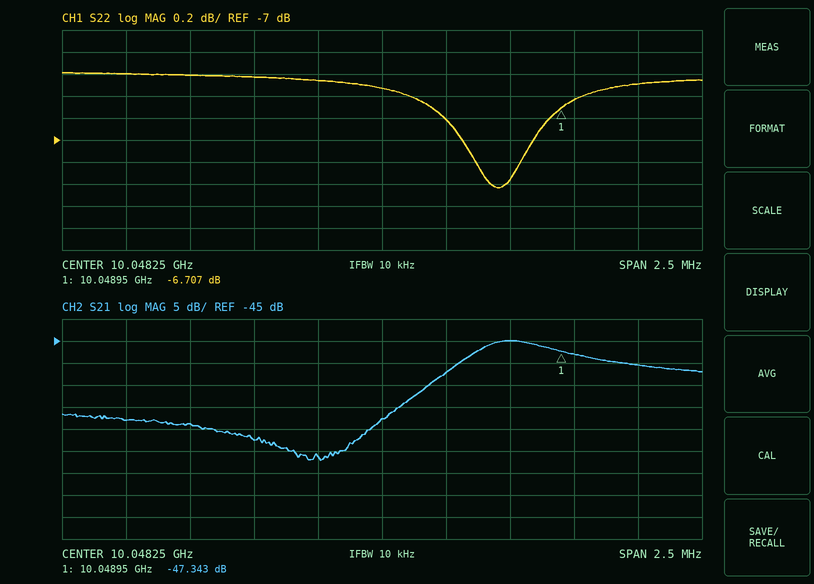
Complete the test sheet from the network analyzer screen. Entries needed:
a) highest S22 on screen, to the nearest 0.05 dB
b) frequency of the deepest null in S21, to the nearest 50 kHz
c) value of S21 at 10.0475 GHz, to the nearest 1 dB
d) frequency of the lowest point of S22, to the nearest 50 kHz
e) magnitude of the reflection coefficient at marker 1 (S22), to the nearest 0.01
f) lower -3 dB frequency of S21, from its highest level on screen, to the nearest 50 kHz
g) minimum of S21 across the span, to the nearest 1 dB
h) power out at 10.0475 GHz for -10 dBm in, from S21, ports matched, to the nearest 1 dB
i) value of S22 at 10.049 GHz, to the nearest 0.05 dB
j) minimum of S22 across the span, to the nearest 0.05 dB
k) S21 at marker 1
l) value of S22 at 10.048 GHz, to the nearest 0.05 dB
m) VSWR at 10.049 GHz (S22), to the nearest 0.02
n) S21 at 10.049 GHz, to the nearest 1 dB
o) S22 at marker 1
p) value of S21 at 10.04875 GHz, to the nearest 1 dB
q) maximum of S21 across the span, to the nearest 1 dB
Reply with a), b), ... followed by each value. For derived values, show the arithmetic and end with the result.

a) -6.40 dB
b) 10.04800 GHz
c) -64 dB
d) 10.04870 GHz
e) 10^(-6.707/20) ≈ 0.46
f) 10.04860 GHz
g) -72 dB
h) -10 dBm + (-64 dB) = -74 dBm
i) -6.65 dB
j) -7.45 dB
k) -47.343 dB
l) -6.45 dB
m) |Γ| = 10^(-6.65/20) = 0.4651; VSWR = (1 + 0.4651)/(1 − 0.4651) ≈ 2.74
n) -48 dB
o) -6.707 dB
p) -45 dB
q) -45 dB
